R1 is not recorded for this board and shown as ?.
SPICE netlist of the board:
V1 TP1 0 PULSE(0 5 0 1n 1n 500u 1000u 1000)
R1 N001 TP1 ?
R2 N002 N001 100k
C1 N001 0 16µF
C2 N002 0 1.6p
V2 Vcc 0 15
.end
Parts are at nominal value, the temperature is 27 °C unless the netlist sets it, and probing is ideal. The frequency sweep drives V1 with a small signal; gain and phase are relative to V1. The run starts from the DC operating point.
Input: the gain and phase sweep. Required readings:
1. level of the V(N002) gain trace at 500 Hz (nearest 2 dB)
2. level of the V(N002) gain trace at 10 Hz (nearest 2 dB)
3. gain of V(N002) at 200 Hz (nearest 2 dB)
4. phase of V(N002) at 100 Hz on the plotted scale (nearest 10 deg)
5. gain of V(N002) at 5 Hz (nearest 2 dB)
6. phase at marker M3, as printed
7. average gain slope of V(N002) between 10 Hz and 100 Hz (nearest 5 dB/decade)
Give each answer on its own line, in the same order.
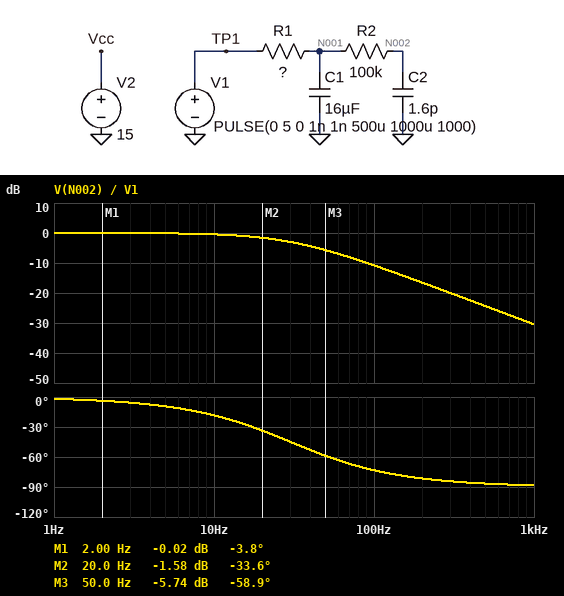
-24 dB
0 dB
-16 dB
-70 deg
0 dB
-58.9 deg
-10 dB/decade
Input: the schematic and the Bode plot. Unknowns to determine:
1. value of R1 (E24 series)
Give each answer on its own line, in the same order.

330 Ω
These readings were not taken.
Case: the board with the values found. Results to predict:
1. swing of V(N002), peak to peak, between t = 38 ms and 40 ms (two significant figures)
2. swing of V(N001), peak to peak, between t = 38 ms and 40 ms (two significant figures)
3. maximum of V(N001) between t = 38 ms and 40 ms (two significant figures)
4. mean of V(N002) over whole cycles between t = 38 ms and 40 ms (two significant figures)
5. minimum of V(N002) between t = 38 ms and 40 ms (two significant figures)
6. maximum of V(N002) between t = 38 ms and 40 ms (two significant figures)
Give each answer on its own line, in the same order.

240 mV
240 mV
2.6 V
2.5 V
2.4 V
2.6 V
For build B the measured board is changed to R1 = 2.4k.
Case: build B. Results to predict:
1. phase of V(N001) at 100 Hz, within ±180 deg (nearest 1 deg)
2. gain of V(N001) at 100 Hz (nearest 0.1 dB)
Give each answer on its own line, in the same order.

-88 deg
-27.7 dB
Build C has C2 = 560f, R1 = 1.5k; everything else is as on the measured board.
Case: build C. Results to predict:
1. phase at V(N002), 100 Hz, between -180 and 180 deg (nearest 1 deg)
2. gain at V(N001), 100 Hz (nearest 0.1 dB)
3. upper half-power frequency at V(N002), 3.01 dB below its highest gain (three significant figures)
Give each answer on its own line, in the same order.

-86 deg
-23.6 dB
6.63 Hz
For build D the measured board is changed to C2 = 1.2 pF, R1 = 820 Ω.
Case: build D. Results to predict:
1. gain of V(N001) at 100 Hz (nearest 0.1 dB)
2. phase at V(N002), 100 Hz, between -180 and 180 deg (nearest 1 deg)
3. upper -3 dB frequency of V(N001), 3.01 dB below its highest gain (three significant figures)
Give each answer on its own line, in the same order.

-18.4 dB
-83 deg
12.1 Hz
